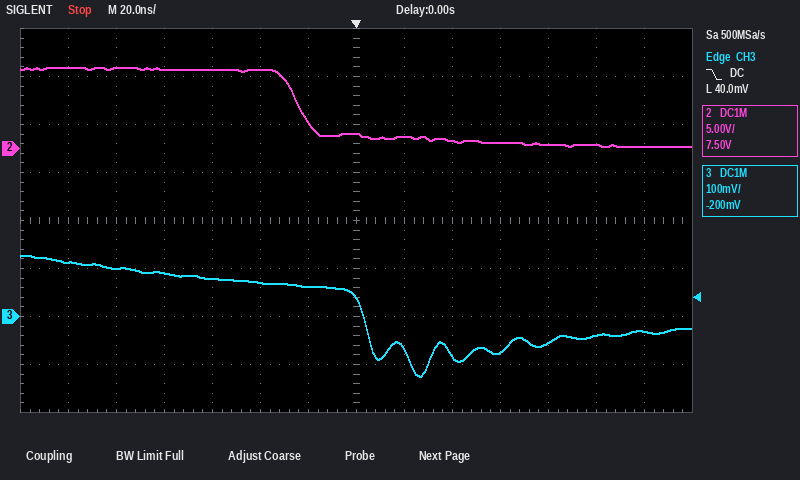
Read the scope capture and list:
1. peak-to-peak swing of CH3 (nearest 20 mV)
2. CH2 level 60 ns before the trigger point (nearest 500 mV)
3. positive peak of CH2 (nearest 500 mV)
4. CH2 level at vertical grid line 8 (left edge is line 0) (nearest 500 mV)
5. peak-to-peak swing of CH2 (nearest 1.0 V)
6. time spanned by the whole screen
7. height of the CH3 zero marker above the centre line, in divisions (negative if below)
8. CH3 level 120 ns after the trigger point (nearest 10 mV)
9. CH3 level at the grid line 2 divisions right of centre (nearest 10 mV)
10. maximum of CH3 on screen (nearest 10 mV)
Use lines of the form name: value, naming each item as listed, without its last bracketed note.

peak-to-peak swing of CH3: 260 mV
CH2 level 60 ns before the trigger point: 8.0 V
positive peak of CH2: 8.5 V
CH2 level at vertical grid line 8 (left edge is line 0): 1.0 V
peak-to-peak swing of CH2: 8.0 V
time spanned by the whole screen: 280 ns
height of the CH3 zero marker above the centre line, in divisions: -2.0 div
CH3 level 120 ns after the trigger point: -30 mV
CH3 level at the grid line 2 divisions right of centre: -80 mV
maximum of CH3 on screen: 130 mV
